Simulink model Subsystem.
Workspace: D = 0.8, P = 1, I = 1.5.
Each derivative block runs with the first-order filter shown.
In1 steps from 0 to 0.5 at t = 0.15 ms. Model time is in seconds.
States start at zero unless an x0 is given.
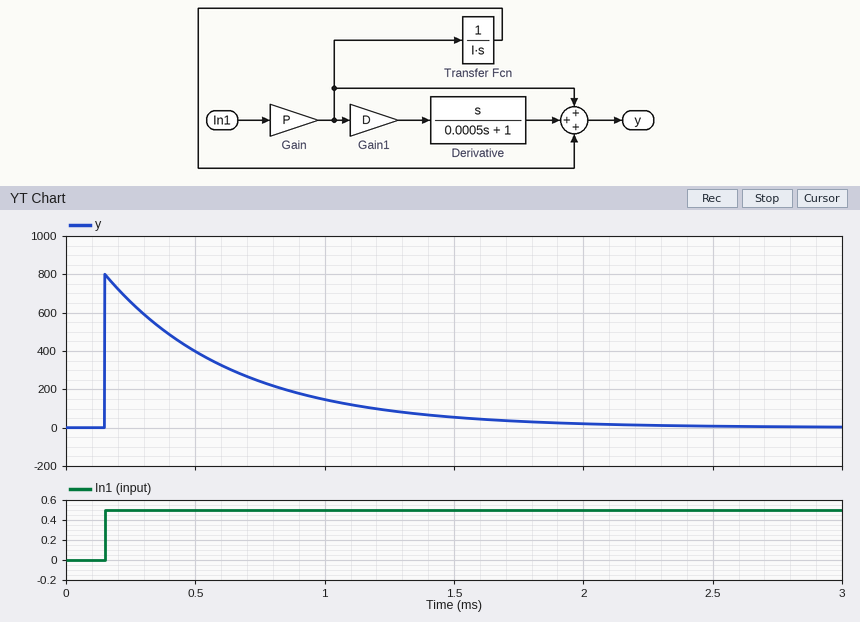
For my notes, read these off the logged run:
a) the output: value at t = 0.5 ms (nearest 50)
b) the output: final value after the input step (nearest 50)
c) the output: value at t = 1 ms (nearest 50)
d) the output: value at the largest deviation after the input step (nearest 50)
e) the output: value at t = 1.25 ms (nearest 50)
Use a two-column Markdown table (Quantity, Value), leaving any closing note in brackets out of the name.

| Quantity | Value |
|---|---|
| the output: value at t = 0.5 ms | 400 |
| the output: final value after the input step | 0 |
| the output: value at t = 1 ms | 150 |
| the output: value at the largest deviation after the input step | 800 |
| the output: value at t = 1.25 ms | 100 |
